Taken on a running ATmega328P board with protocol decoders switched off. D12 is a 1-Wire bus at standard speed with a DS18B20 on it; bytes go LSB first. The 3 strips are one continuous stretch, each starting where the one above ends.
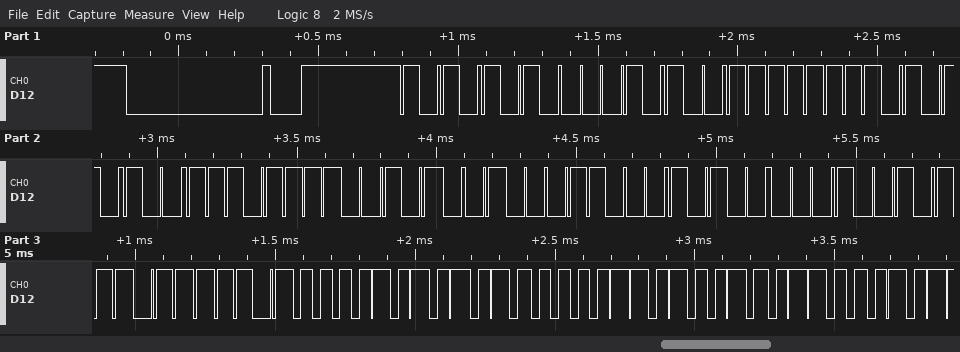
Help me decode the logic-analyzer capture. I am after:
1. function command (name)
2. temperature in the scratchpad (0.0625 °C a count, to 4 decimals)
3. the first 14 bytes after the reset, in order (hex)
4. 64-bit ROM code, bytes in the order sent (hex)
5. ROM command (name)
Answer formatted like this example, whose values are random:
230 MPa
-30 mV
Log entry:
Read Scratchpad
85.0000 °C
55 28 FF 2A F7 94 18 05 E9 BE 50 05 4B 46
28 FF 2A F7 94 18 05 E9
Match ROM
